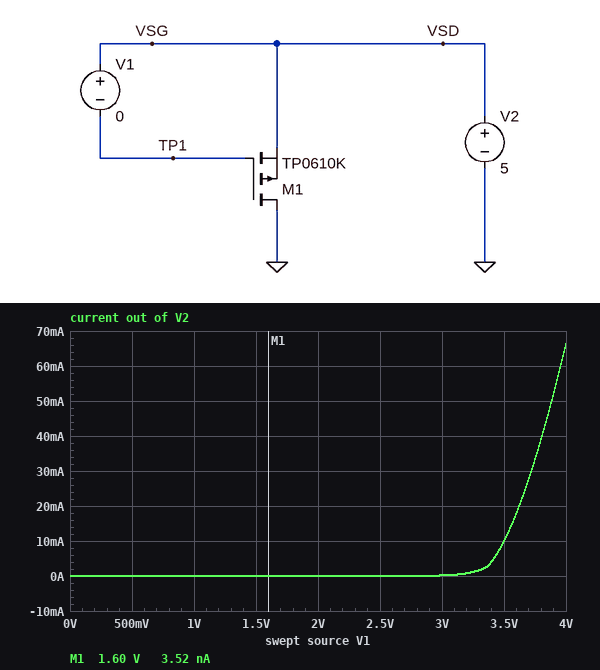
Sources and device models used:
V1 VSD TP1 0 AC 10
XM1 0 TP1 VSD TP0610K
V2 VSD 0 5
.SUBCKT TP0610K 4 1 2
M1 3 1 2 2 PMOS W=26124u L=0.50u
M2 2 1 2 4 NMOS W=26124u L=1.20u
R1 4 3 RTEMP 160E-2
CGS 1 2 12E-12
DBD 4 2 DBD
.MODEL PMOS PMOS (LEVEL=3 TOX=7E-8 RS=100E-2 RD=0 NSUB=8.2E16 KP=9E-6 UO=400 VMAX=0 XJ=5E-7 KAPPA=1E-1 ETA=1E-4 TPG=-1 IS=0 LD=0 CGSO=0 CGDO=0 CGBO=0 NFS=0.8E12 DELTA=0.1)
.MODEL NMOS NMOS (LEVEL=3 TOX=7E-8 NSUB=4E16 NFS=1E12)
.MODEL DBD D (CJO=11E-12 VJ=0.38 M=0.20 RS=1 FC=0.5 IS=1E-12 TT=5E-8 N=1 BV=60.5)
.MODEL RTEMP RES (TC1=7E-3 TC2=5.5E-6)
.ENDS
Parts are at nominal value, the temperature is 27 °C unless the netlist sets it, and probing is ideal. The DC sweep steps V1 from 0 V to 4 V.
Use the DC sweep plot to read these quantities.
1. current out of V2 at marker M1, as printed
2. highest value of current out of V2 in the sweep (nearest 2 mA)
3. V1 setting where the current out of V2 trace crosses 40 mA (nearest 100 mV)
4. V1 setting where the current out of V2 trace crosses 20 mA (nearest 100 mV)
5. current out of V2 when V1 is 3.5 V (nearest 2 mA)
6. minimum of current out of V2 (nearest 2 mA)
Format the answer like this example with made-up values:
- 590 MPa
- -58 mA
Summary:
- 3.52 nA
- 66 mA
- 3.8 V
- 3.6 V
- 10 mA
- 0 A
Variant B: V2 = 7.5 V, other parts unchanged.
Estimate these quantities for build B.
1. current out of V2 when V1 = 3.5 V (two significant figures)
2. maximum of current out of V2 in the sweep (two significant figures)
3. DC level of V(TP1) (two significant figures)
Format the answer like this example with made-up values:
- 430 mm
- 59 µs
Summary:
- 11 mA
- 69 mA
- 7.5 V
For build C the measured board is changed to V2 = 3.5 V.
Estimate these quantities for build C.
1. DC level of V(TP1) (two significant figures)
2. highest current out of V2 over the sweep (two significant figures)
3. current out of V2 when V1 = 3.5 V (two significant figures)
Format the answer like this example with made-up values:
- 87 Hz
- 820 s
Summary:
- 3.5 V
- 64 mA
- 9.5 mA
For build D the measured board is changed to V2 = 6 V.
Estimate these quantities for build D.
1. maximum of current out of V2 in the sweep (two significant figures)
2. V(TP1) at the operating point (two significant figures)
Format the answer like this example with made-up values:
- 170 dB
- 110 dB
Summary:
- 68 mA
- 6.0 V
